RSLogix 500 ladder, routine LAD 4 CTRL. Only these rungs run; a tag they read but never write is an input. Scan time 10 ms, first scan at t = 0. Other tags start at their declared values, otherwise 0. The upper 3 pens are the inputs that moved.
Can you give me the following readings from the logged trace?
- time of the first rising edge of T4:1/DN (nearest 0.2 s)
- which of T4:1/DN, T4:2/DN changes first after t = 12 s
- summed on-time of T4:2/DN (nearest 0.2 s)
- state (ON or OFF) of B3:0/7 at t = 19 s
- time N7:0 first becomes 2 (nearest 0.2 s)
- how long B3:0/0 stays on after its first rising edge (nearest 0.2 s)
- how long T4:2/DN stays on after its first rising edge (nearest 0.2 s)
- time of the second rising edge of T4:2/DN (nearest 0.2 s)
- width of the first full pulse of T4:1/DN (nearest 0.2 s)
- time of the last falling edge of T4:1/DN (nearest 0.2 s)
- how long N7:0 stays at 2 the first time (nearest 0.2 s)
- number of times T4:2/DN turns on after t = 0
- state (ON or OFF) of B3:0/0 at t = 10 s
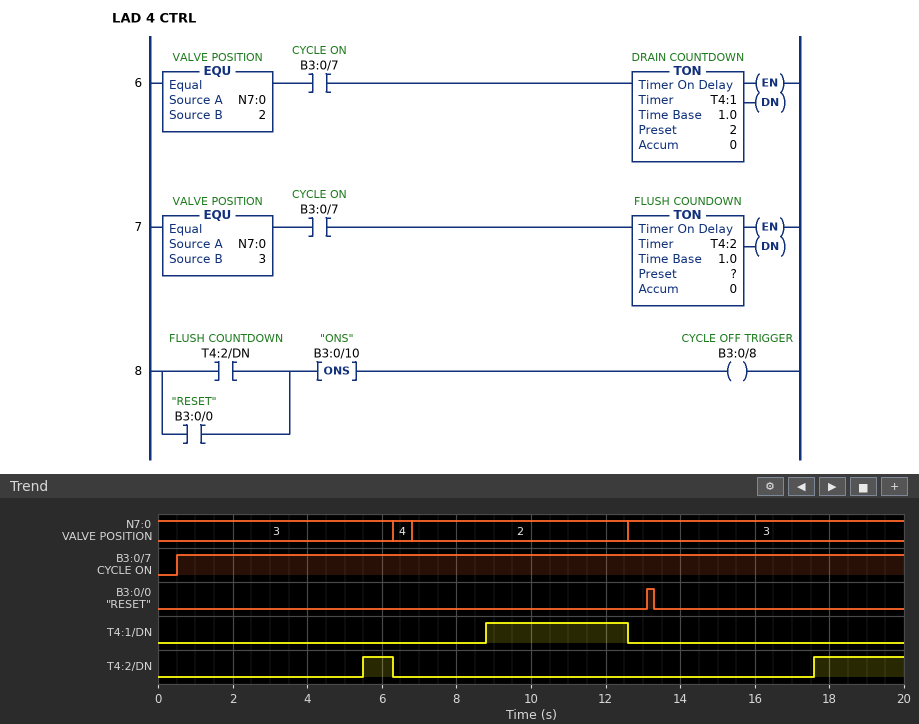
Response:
8.8 s
T4:1/DN
3.2 s
ON
6.8 s
0.2 s
0.8 s
17.6 s
3.8 s
12.6 s
5.8 s
2
OFF
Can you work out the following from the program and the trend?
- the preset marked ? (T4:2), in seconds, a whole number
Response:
5 s
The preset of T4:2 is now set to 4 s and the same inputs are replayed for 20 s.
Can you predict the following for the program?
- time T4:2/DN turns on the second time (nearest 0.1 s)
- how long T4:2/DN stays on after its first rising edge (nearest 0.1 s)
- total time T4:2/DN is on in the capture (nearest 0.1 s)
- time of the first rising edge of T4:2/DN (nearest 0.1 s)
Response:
16.6 s
1.8 s
5.2 s
4.5 s
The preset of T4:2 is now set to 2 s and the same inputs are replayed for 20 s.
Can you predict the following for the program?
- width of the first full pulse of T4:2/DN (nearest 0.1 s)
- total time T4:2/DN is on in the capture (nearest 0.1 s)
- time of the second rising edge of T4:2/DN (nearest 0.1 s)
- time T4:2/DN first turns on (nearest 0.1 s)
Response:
3.8 s
9.2 s
14.6 s
2.5 s
